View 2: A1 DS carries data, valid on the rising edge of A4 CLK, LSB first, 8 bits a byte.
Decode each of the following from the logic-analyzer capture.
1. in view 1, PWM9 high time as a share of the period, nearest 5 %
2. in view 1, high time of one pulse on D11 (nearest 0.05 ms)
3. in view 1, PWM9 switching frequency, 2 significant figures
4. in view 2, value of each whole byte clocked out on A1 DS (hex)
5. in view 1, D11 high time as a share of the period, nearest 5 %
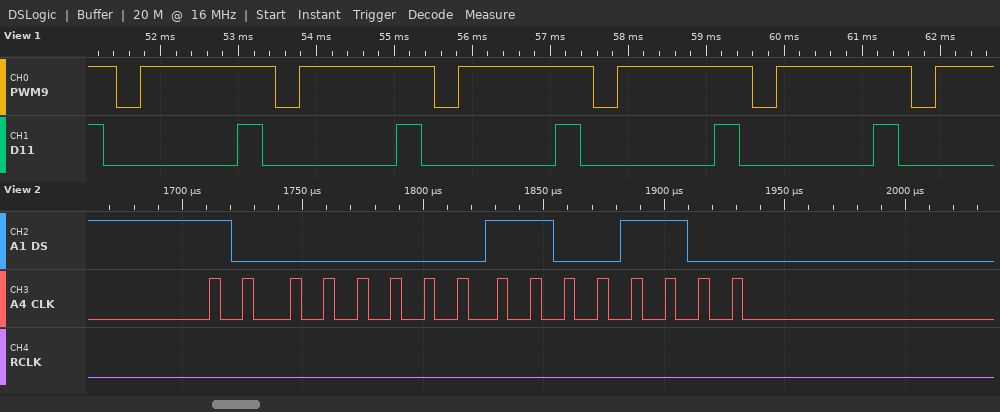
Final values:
85 %
0.30 ms
490 Hz
01 33
15 %
